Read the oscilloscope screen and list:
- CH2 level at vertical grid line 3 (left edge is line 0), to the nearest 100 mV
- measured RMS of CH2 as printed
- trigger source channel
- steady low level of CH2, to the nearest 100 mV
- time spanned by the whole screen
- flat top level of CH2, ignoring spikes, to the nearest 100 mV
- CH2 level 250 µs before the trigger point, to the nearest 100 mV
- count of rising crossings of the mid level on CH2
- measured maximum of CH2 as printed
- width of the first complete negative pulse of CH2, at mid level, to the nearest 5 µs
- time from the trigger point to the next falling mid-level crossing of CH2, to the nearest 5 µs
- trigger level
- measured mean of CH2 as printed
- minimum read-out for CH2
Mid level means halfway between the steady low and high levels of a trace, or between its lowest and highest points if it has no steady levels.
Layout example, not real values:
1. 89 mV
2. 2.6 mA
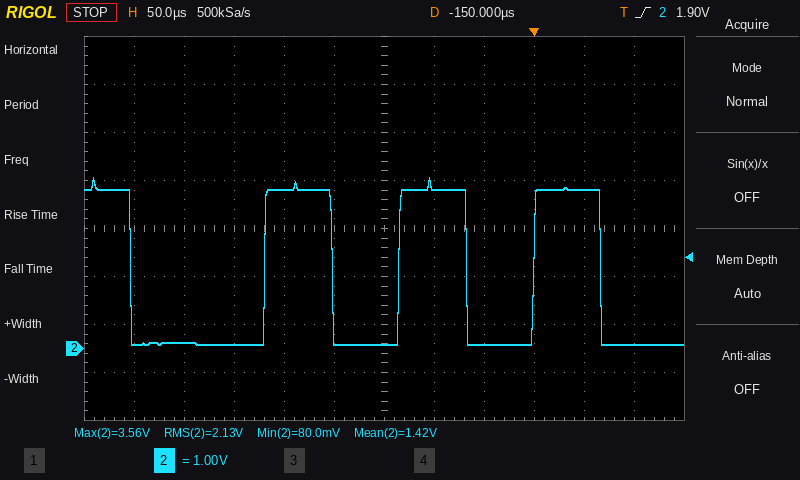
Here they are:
1. 100 mV
2. 2.13 V
3. CH2
4. 100 mV
5. 600 µs
6. 3.3 V
7. 3.3 V
8. 3
9. 3.56 V
10. 135 µs
11. 65 µs
12. 1.90 V
13. 1.42 V
14. 80.0 mV
